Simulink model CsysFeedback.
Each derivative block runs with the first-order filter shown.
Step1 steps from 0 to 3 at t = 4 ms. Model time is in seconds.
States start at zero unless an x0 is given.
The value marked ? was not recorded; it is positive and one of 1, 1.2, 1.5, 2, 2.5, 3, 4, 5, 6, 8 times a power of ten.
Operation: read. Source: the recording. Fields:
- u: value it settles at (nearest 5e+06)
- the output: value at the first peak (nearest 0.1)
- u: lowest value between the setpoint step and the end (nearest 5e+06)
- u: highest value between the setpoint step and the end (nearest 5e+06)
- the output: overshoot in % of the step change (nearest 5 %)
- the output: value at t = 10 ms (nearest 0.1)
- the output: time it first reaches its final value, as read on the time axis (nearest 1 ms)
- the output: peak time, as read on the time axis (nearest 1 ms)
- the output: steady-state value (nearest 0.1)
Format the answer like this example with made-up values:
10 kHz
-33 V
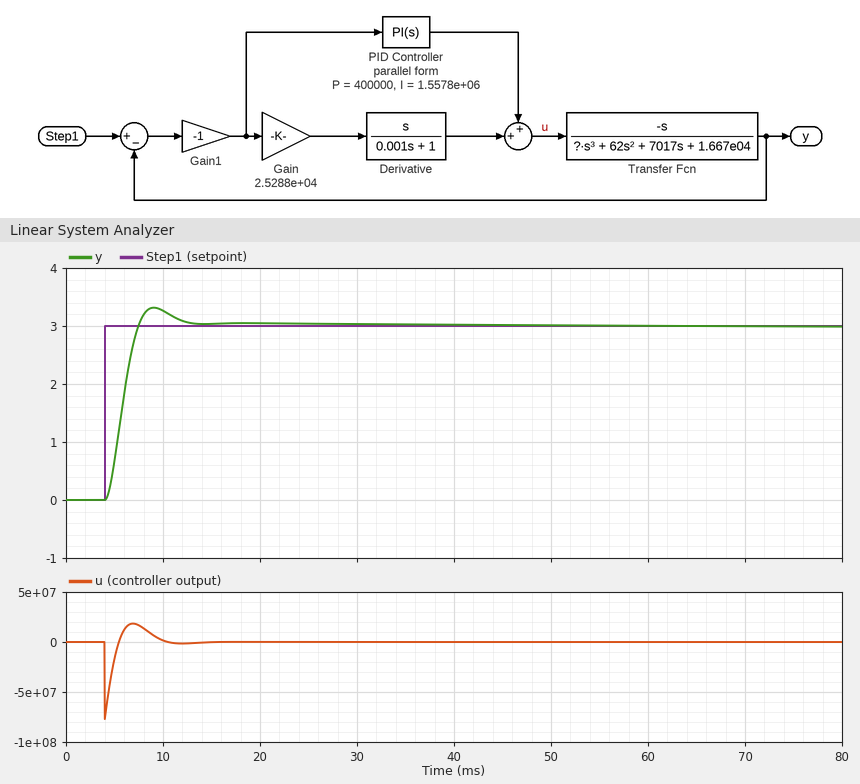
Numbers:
0
3.3
-75000000
20000000
10 %
3.3
7 ms
9 ms
3.0
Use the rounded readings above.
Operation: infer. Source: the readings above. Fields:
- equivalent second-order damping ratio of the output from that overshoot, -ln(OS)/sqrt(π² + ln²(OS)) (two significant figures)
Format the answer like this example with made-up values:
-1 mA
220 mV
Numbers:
0.59
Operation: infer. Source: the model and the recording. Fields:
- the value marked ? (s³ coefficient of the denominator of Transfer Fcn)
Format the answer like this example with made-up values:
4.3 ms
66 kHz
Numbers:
40
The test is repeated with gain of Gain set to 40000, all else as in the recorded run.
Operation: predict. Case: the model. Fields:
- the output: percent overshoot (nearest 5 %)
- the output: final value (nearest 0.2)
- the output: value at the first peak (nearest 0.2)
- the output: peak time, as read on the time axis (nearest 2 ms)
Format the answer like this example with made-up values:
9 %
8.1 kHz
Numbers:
20 %
3.0
3.6
8 ms
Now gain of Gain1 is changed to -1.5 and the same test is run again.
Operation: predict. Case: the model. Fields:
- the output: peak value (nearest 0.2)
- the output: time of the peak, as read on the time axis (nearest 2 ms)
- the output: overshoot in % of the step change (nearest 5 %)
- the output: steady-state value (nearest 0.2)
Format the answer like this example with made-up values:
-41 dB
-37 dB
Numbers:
3.6
8 ms
20 %
3.0
